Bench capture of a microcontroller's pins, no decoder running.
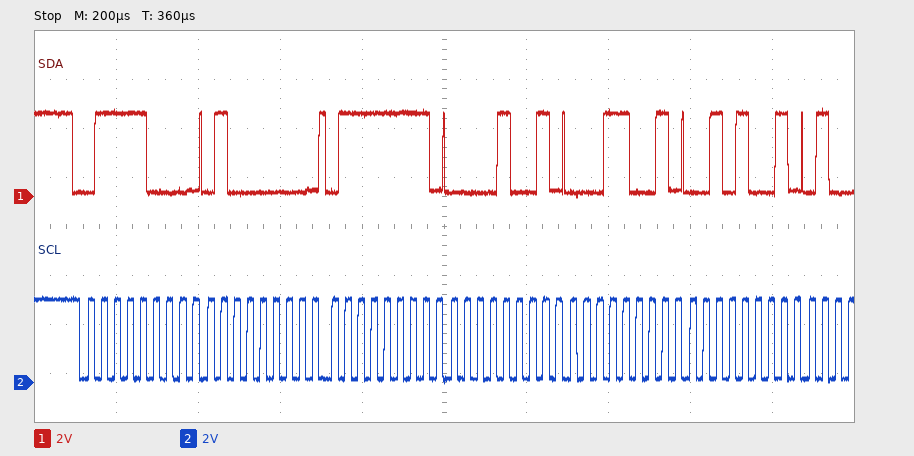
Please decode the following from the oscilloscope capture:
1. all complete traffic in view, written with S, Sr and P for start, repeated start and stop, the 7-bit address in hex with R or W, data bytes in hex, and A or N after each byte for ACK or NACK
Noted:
S 3CW A 40 A 7F A 09 A 19 A 29 A
